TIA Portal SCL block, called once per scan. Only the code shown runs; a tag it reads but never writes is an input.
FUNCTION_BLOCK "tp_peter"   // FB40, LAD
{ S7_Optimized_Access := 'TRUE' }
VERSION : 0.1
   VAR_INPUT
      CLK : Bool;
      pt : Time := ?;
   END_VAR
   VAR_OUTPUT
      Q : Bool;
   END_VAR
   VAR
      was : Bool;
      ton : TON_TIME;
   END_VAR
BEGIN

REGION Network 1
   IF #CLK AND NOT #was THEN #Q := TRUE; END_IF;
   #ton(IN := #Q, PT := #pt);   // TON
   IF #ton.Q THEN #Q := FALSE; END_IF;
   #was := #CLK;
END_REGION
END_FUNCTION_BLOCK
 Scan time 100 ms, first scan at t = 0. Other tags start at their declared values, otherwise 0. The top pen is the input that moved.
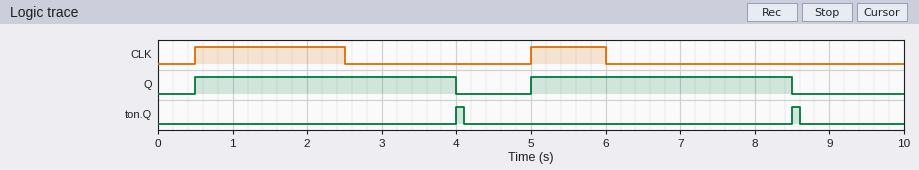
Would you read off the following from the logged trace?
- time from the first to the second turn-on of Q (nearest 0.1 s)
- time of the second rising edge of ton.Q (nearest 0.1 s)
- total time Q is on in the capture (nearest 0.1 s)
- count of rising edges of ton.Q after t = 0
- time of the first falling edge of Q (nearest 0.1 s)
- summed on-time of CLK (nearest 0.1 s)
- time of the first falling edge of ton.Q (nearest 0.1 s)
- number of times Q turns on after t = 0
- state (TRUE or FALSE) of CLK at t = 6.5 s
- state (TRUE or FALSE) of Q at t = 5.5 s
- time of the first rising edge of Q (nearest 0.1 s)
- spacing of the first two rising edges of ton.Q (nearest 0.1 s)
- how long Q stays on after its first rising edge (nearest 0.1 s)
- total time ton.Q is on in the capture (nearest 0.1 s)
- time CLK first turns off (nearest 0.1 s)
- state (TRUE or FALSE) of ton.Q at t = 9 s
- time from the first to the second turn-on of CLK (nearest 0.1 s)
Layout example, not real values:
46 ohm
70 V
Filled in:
4.5 s
8.5 s
7.0 s
2
4.0 s
3.0 s
4.1 s
2
FALSE
TRUE
0.5 s
4.5 s
3.5 s
0.2 s
2.5 s
FALSE
4.5 s
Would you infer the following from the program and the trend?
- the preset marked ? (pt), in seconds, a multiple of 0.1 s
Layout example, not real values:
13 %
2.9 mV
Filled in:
3.5 s
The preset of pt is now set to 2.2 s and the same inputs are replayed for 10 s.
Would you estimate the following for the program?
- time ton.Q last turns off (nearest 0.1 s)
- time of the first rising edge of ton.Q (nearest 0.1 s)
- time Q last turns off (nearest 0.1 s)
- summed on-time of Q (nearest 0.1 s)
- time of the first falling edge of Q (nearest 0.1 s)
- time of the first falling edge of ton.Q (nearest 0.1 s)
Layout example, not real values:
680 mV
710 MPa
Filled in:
7.3 s
2.7 s
7.2 s
4.4 s
2.7 s
2.8 s
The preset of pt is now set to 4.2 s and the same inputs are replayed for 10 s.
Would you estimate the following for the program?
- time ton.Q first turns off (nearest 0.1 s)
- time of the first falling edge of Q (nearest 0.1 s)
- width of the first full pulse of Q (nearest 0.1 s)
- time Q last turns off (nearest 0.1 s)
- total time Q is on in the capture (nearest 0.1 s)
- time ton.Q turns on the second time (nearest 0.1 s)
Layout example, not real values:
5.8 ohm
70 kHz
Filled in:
4.8 s
4.7 s
4.2 s
9.2 s
8.4 s
9.2 s
